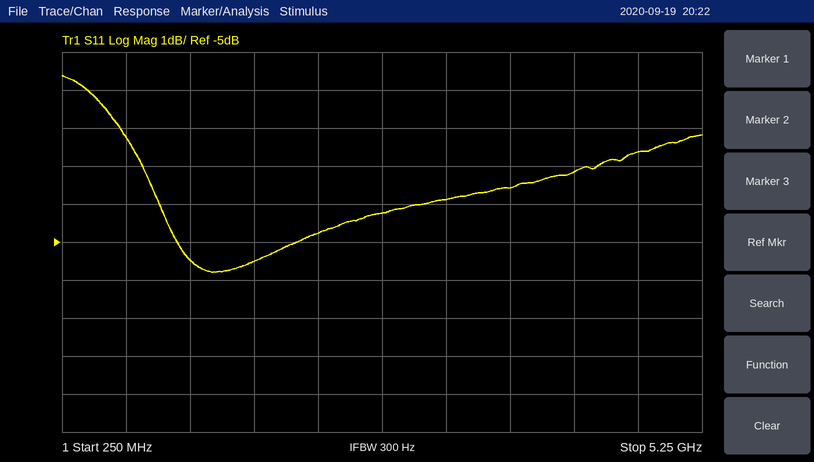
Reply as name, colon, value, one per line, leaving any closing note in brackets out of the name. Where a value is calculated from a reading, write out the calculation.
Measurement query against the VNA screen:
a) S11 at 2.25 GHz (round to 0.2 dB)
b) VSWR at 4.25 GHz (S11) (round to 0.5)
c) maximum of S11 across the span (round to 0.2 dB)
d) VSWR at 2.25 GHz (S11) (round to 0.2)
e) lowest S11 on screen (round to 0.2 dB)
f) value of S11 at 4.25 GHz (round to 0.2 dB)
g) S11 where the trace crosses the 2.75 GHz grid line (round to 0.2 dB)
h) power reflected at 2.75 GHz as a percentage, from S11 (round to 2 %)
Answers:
S11 at 2.25 GHz: -4.8 dB
VSWR at 4.25 GHz (S11): |Γ| = 10^(-3.2/20) = 0.6918; VSWR = (1 + 0.6918)/(1 − 0.6918) ≈ 5.5
maximum of S11 across the span: -0.6 dB
VSWR at 2.25 GHz (S11): |Γ| = 10^(-4.8/20) = 0.5754; VSWR = (1 + 0.5754)/(1 − 0.5754) ≈ 3.71, so 3.8 to the nearest 0.2
lowest S11 on screen: -5.8 dB
value of S11 at 4.25 GHz: -3.2 dB
S11 where the trace crosses the 2.75 GHz grid line: -4.2 dB
power reflected at 2.75 GHz as a percentage, from S11: 10^(-4.2/10) ≈ 38 %
